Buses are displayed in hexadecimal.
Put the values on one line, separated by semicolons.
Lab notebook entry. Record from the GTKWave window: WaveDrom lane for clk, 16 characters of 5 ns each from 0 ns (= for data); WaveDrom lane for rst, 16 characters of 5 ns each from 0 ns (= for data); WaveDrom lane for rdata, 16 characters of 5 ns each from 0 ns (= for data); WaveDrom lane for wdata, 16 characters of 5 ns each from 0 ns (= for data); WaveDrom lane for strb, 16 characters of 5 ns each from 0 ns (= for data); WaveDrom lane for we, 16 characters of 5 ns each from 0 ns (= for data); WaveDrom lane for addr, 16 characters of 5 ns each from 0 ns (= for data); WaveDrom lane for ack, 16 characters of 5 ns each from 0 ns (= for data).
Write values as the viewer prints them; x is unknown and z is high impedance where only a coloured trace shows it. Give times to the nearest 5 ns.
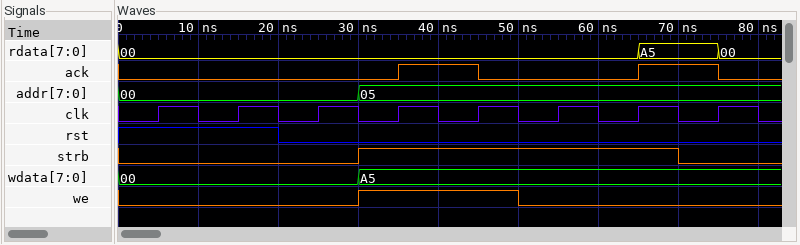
{name: 'clk', wave: '0101010101010101'}; {name: 'rst', wave: '1...0...........'}; {name: 'rdata', wave: '=............=.=', data: '00 A5 00'}; {name: 'wdata', wave: '=.....=.........', data: '00 A5'}; {name: 'strb', wave: '0.....1.......0.'}; {name: 'we', wave: '0.....1...0.....'}; {name: 'addr', wave: '=.....=.........', data: '00 05'}; {name: 'ack', wave: '0......1.0...1.0'}
